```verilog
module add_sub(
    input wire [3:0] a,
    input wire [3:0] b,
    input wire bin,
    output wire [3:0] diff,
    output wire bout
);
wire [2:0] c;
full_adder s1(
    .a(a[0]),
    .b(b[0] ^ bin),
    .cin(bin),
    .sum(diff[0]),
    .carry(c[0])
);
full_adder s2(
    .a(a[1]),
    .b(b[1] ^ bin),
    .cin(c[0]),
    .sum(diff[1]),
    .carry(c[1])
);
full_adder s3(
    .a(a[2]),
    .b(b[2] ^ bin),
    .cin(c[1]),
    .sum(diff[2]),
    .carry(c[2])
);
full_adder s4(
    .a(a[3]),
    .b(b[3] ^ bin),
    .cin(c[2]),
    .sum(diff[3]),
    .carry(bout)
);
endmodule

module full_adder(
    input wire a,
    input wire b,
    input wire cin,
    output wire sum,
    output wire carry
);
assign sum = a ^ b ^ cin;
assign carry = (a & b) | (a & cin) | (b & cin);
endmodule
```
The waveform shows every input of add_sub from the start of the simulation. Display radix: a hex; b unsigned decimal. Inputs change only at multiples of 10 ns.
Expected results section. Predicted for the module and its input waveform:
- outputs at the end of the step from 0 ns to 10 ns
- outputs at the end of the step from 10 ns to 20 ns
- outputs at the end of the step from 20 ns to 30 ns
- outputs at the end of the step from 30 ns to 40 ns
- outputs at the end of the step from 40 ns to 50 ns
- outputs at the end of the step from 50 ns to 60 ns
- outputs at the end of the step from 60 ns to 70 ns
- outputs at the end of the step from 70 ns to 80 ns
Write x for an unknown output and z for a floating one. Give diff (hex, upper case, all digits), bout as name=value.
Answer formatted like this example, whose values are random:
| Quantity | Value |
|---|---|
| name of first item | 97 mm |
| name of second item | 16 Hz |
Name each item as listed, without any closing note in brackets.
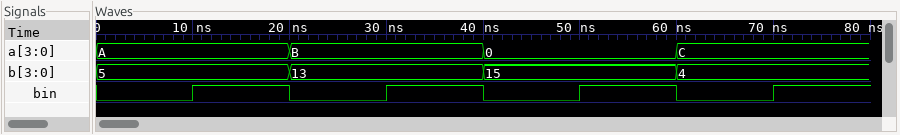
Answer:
| Quantity | Value |
|---|---|
| outputs at the end of the step from 0 ns to 10 ns | diff=F, bout=0 |
| outputs at the end of the step from 10 ns to 20 ns | diff=5, bout=1 |
| outputs at the end of the step from 20 ns to 30 ns | diff=8, bout=1 |
| outputs at the end of the step from 30 ns to 40 ns | diff=E, bout=0 |
| outputs at the end of the step from 40 ns to 50 ns | diff=F, bout=0 |
| outputs at the end of the step from 50 ns to 60 ns | diff=1, bout=0 |
| outputs at the end of the step from 60 ns to 70 ns | diff=0, bout=1 |
| outputs at the end of the step from 70 ns to 80 ns | diff=8, bout=1 |
